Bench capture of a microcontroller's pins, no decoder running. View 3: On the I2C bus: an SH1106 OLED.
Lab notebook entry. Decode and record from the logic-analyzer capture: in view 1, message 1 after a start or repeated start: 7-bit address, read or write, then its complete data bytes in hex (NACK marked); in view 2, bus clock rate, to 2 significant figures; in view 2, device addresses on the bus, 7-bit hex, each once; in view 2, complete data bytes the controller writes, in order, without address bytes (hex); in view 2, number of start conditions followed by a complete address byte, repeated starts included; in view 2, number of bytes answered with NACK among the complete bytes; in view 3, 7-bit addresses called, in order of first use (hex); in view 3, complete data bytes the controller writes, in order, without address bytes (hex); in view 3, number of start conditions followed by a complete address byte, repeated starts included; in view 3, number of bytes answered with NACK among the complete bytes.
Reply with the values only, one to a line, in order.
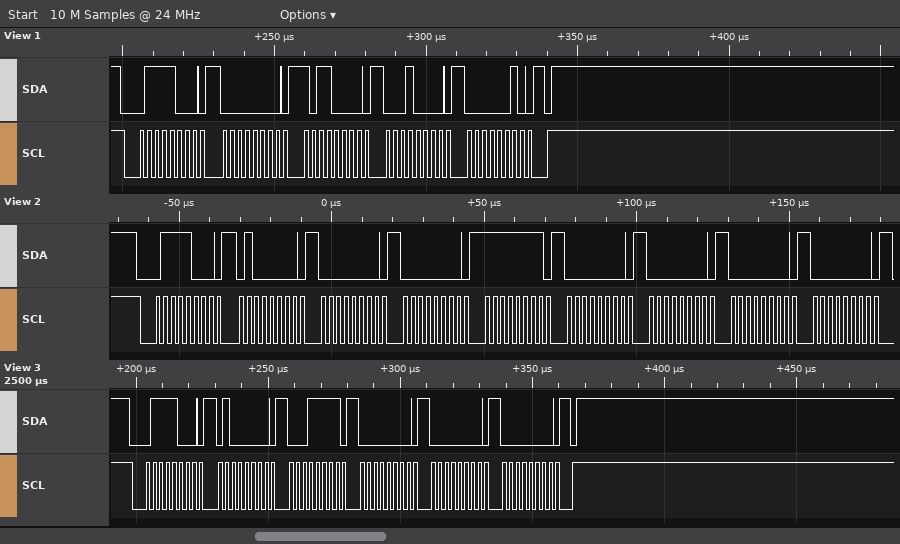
0x3C write: 00 B0 10 02
400 kHz
0x3C
40 00 00 FF 00 00 00 00
1
0
0x3C
40 1F 00 00 00
1
0
